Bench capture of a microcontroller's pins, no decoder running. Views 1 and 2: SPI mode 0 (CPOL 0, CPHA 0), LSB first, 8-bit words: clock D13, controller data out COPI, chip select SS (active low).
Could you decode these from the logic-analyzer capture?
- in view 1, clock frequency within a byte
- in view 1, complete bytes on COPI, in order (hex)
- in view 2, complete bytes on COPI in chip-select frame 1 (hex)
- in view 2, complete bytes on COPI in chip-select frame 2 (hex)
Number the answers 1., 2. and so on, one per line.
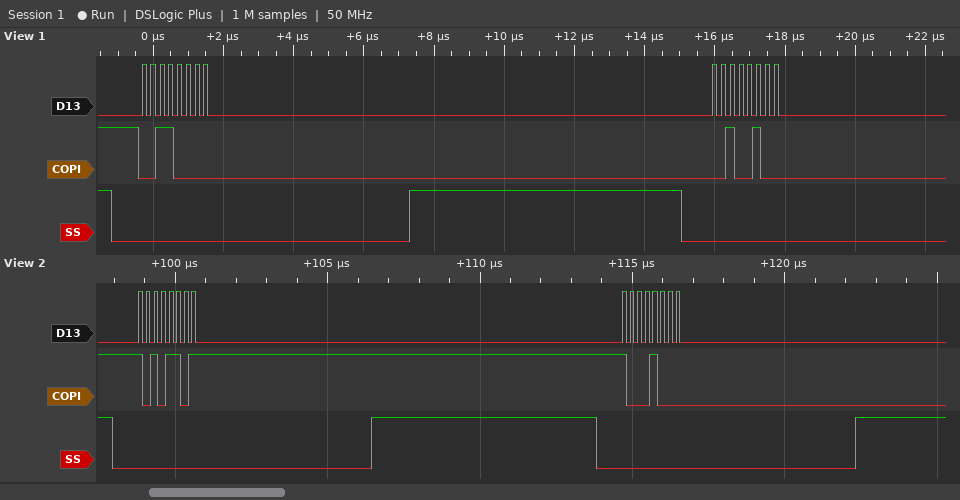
1. 4 MHz
2. 0x0C 0x24
3. 0xB5
4. 0x11
